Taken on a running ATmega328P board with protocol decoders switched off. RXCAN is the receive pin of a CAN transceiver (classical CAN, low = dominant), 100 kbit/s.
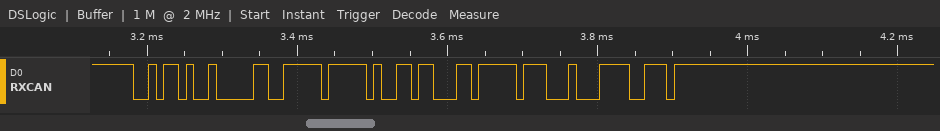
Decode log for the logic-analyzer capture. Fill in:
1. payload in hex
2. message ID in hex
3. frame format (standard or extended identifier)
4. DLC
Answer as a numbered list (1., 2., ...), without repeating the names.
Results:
1. FF E6 C6 FF
2. 0x2D2
3. standard
4. 4
